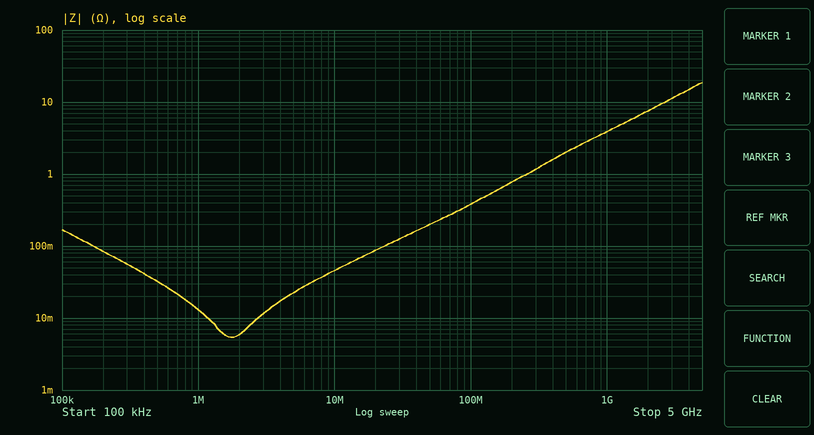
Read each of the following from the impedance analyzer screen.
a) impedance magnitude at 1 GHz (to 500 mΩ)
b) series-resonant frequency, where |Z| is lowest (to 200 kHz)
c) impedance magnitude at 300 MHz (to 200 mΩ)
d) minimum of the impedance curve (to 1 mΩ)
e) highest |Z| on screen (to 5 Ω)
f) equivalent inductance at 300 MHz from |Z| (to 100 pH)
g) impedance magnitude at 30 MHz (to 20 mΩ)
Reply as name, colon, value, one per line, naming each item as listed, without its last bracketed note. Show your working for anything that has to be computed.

impedance magnitude at 1 GHz: 4.0 Ω
series-resonant frequency, where |Z| is lowest: 1.8 MHz
impedance magnitude at 300 MHz: 1.2 Ω
minimum of the impedance curve: 5 mΩ
highest |Z| on screen: 20 Ω
equivalent inductance at 300 MHz from |Z|: L = 1.2 Ω/(2π × 300 MHz) ≈ 637 pH, so 600 pH to the nearest 100 pH
impedance magnitude at 30 MHz: 120 mΩ
